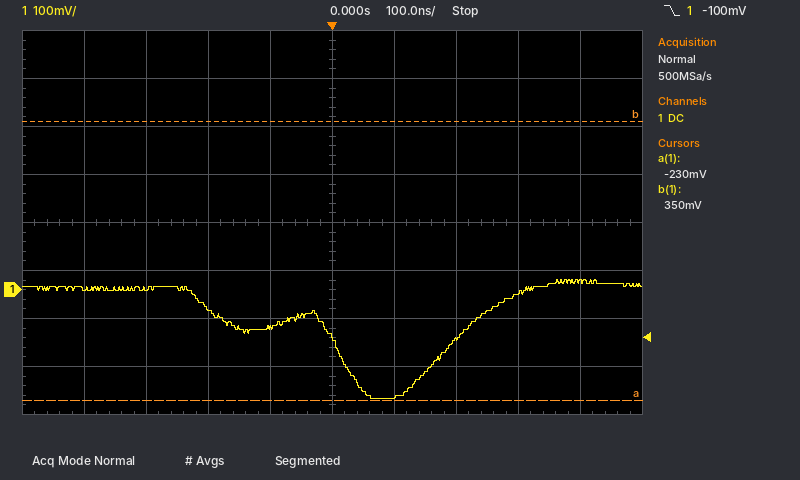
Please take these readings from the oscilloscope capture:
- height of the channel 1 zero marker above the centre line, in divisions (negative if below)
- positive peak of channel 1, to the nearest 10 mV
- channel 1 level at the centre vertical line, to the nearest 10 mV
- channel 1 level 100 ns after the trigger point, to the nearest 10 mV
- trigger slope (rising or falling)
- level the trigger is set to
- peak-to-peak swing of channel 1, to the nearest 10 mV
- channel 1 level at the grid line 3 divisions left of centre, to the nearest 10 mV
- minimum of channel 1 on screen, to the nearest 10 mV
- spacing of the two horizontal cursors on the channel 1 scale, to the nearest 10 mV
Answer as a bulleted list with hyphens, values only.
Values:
- -1.4 div
- 20 mV
- -100 mV
- -220 mV
- falling
- -100 mV
- 250 mV
- 0 mV
- -230 mV
- 580 mV
